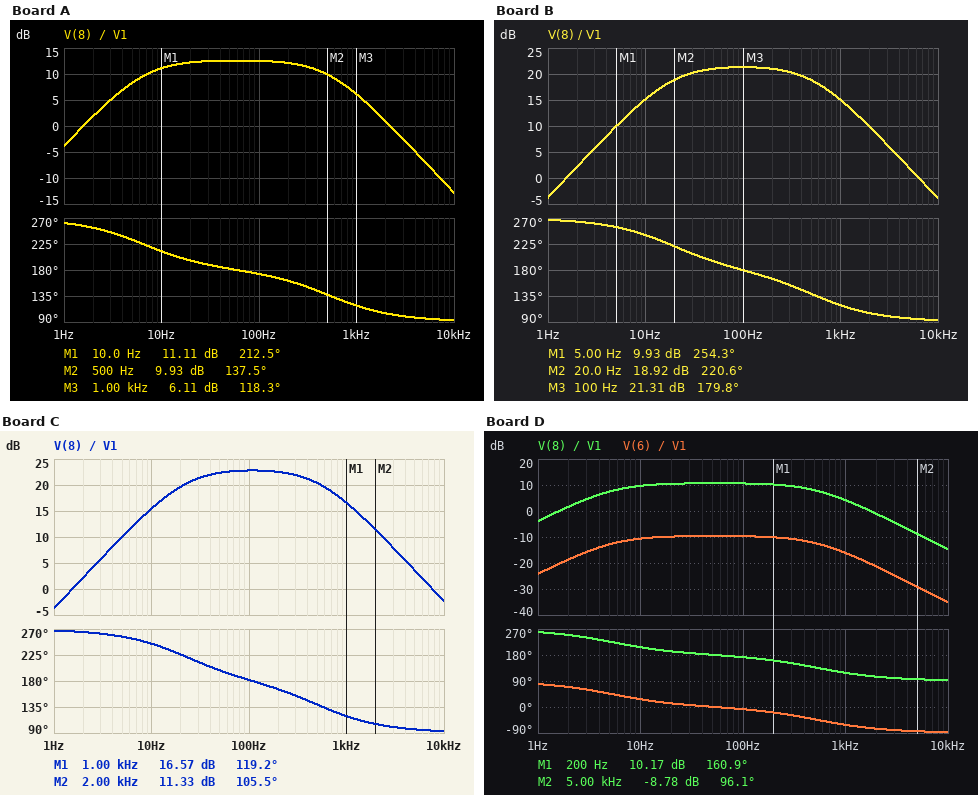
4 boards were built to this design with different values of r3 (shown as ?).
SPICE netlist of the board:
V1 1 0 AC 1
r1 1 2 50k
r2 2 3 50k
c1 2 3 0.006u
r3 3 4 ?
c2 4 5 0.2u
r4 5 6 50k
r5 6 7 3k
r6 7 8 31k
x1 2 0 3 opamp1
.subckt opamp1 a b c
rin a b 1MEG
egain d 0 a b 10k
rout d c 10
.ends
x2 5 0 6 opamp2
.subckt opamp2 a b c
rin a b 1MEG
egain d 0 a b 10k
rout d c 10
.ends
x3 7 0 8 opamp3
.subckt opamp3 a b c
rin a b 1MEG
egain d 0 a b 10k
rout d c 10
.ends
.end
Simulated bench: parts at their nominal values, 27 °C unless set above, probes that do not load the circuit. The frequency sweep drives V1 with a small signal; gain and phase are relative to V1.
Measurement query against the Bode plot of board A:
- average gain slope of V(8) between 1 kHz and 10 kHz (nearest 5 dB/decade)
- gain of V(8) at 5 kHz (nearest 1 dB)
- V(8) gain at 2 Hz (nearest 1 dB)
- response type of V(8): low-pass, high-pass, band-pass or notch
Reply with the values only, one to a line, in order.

-20 dB/decade
-7 dB
2 dB
band-pass
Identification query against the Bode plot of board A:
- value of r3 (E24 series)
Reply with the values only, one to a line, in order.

120 kΩ
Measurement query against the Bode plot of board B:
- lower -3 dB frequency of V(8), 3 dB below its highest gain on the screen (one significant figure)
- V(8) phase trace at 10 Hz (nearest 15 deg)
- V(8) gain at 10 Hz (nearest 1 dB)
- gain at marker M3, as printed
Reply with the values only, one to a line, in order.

20 Hz
240 deg
15 dB
21.31 dB
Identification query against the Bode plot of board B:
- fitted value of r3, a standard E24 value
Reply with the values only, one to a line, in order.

43 kΩ
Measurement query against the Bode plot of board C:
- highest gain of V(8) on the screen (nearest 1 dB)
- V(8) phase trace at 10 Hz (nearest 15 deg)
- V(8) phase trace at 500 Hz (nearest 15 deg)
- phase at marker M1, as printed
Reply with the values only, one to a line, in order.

23 dB
240 deg
135 deg
119.2 deg
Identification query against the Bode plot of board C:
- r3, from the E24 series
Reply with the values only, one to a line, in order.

36 kΩ
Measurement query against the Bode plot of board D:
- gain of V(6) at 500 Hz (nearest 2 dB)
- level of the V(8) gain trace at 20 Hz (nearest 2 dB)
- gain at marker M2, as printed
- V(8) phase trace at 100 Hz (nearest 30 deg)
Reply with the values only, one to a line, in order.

-12 dB
10 dB
-8.78 dB
180 deg
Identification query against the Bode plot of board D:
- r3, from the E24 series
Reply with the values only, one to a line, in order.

150 kΩ
